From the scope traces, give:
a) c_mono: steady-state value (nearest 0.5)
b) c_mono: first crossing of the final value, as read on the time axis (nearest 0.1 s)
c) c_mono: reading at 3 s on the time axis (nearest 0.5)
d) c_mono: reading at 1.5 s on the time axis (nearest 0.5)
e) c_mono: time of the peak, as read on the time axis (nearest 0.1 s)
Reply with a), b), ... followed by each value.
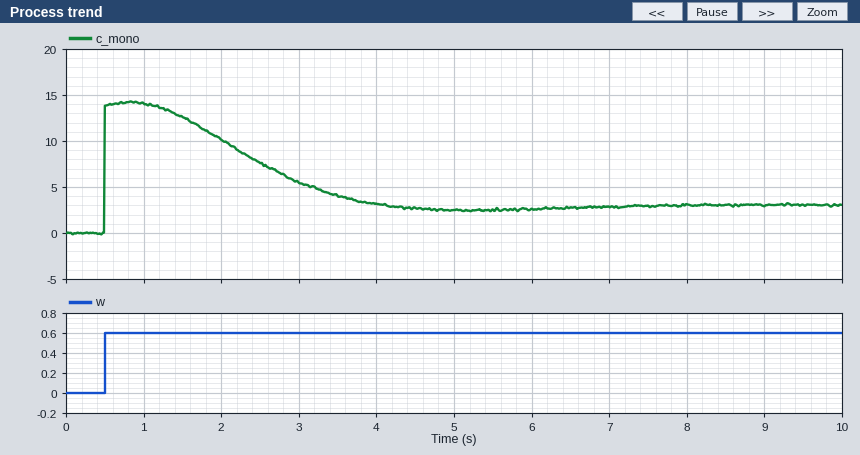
a) 3.0
b) 0.5 s
c) 5.5
d) 12.5
e) 0.8 s
